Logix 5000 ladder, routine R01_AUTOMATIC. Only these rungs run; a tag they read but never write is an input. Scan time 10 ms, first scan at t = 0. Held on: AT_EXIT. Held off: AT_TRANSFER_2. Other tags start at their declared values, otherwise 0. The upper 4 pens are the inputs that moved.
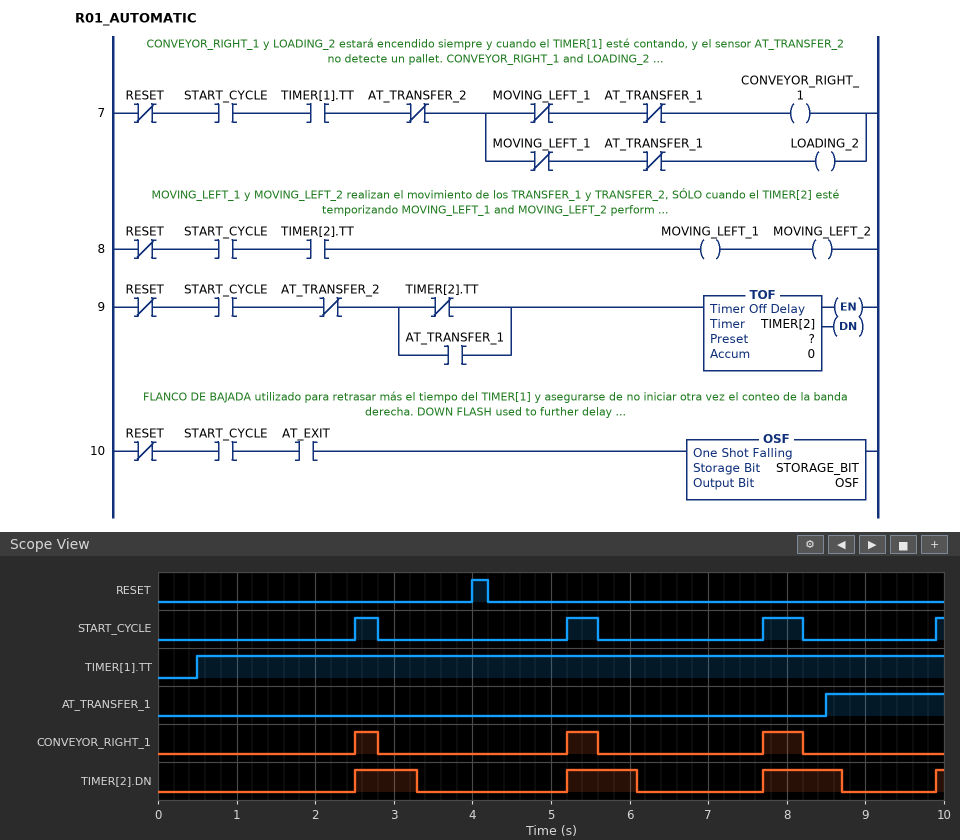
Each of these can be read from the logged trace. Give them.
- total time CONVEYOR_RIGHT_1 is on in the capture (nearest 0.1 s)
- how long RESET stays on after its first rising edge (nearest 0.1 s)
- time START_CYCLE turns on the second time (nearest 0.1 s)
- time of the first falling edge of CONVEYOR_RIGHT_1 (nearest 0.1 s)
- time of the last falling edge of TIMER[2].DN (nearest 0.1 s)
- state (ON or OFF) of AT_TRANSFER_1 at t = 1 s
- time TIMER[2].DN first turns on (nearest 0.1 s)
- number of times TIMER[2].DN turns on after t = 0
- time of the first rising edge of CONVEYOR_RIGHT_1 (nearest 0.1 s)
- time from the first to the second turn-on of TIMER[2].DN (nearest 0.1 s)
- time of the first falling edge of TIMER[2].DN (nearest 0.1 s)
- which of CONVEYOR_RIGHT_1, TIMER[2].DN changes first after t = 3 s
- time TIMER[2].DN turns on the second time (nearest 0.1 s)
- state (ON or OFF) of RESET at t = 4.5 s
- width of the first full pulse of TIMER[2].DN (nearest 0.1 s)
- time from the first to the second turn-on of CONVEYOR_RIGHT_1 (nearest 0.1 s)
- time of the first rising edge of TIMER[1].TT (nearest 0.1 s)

1.2 s
0.2 s
5.2 s
2.8 s
8.7 s
OFF
2.5 s
4
2.5 s
2.7 s
3.3 s
TIMER[2].DN
5.2 s
OFF
0.8 s
2.7 s
0.5 s
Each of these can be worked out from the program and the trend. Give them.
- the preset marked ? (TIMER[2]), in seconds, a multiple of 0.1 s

0.5 s
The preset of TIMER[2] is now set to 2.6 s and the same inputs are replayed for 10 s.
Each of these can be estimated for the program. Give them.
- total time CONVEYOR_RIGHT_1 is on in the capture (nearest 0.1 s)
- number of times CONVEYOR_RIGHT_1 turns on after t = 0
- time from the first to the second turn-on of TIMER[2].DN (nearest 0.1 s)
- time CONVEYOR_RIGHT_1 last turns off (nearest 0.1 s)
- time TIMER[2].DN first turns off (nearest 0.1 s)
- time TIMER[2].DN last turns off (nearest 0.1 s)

0.5 s
4
2.9 s
7.7 s
5.4 s
8.2 s
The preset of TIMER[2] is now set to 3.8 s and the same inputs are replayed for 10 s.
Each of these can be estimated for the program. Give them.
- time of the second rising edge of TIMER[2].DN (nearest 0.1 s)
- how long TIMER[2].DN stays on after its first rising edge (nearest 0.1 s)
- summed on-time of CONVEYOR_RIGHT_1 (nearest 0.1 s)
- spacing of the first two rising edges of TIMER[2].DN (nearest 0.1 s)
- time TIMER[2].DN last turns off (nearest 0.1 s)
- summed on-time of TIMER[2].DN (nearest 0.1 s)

7.7 s
4.1 s
0.8 s
5.2 s
6.6 s
6.4 s
